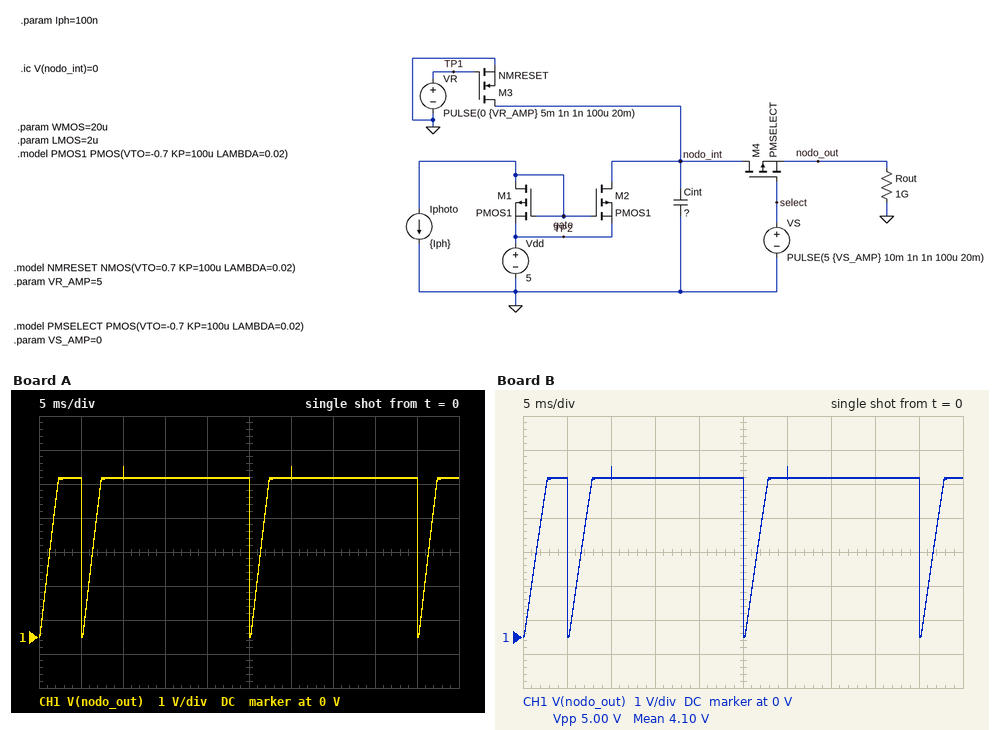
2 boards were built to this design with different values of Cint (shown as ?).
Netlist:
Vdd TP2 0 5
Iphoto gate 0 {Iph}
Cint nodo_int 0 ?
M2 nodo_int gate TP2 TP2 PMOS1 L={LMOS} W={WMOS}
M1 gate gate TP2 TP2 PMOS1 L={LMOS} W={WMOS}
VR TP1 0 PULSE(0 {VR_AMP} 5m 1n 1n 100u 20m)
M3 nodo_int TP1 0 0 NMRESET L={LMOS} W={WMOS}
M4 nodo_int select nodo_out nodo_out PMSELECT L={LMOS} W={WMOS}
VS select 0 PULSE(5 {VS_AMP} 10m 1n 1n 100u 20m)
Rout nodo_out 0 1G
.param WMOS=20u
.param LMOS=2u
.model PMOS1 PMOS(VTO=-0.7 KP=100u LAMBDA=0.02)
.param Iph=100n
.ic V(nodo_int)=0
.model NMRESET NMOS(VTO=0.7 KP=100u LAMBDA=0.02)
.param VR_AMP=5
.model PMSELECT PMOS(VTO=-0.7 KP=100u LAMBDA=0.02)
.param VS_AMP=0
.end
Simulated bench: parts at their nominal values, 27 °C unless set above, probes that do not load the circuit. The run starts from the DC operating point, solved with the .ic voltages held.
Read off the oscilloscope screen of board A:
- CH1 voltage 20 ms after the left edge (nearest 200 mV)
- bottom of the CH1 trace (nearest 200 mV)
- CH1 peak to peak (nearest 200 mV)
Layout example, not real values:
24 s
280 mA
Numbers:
4.6 V
0 V
5.0 V
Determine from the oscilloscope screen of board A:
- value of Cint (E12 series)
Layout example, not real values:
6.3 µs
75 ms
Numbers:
47 pF
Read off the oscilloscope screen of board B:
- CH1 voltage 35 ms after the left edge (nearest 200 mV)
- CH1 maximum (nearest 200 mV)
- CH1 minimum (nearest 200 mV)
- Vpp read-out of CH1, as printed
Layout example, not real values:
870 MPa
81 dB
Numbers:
4.6 V
5.0 V
0 V
5.00 V
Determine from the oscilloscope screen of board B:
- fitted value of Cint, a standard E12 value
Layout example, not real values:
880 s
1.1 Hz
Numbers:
56 pF
